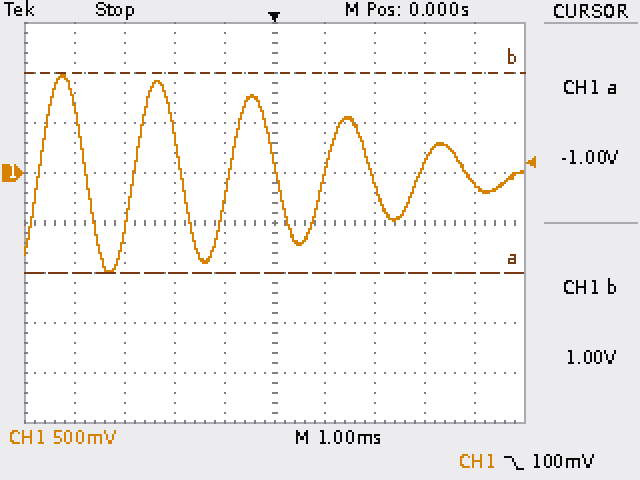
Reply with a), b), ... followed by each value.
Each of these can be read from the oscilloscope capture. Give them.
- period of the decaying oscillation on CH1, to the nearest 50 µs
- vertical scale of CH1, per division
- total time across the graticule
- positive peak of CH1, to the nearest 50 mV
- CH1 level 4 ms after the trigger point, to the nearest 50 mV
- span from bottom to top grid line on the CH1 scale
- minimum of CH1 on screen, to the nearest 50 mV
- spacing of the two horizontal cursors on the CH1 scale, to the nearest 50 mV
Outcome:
a) 1.90 ms
b) 500 mV
c) 10 ms
d) 1.00 V
e) -100 mV
f) 4 V
g) -1.00 V
h) 2.00 V
